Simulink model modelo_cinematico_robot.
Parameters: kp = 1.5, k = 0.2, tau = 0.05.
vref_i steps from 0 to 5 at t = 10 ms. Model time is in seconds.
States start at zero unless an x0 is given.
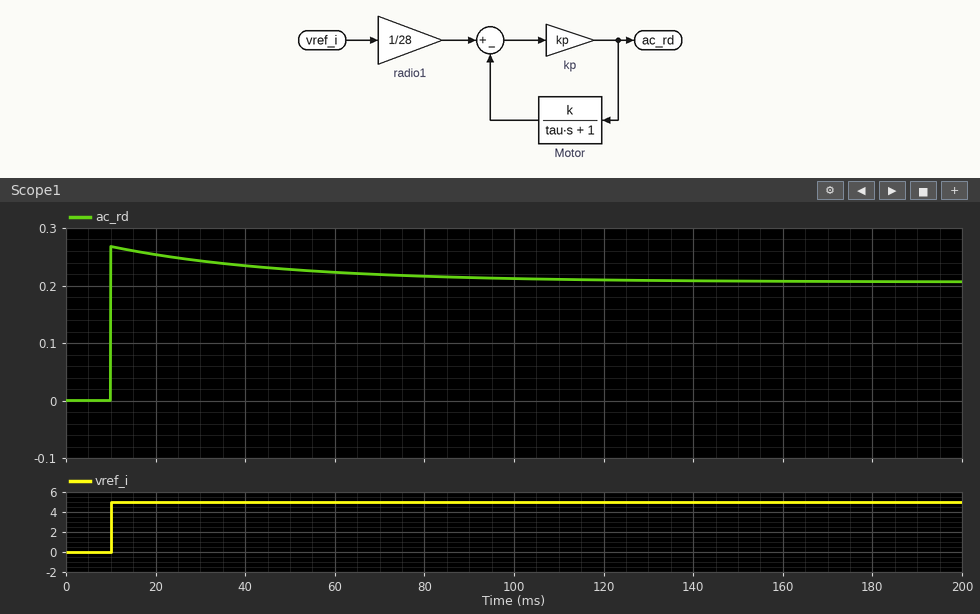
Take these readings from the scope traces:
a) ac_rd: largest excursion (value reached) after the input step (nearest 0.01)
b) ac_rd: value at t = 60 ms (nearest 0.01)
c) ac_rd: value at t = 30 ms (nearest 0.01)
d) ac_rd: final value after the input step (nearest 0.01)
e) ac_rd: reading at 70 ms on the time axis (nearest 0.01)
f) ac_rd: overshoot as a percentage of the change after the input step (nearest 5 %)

0.27
0.22
0.24
0.21
0.22
30 %
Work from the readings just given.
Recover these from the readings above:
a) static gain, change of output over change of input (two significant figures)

0.042
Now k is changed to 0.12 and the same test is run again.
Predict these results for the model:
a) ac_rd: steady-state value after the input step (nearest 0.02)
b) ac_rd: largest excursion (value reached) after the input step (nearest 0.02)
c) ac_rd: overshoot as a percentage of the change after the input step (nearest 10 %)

0.22
0.26
20 %
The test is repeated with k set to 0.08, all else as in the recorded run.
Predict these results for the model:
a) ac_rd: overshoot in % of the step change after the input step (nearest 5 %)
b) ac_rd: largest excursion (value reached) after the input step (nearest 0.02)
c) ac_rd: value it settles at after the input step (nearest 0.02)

10 %
0.26
0.24
